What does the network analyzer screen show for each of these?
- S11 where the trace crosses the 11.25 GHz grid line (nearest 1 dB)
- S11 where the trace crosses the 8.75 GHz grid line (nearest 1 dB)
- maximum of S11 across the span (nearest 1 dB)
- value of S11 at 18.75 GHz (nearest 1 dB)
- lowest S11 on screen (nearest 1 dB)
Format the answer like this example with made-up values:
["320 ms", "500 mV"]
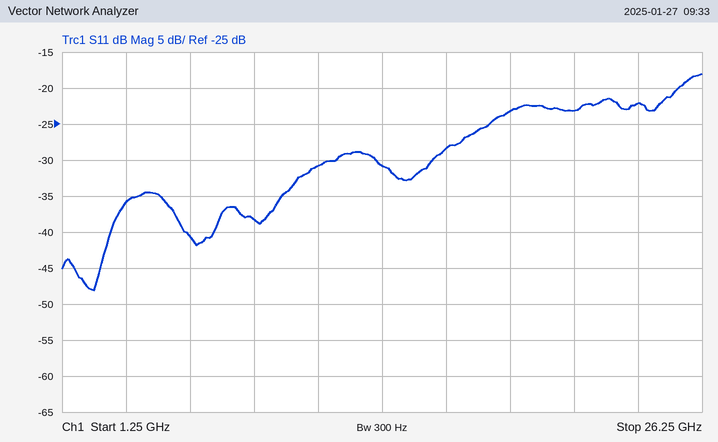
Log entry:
["-31 dB", "-38 dB", "-18 dB", "-23 dB", "-48 dB"]
